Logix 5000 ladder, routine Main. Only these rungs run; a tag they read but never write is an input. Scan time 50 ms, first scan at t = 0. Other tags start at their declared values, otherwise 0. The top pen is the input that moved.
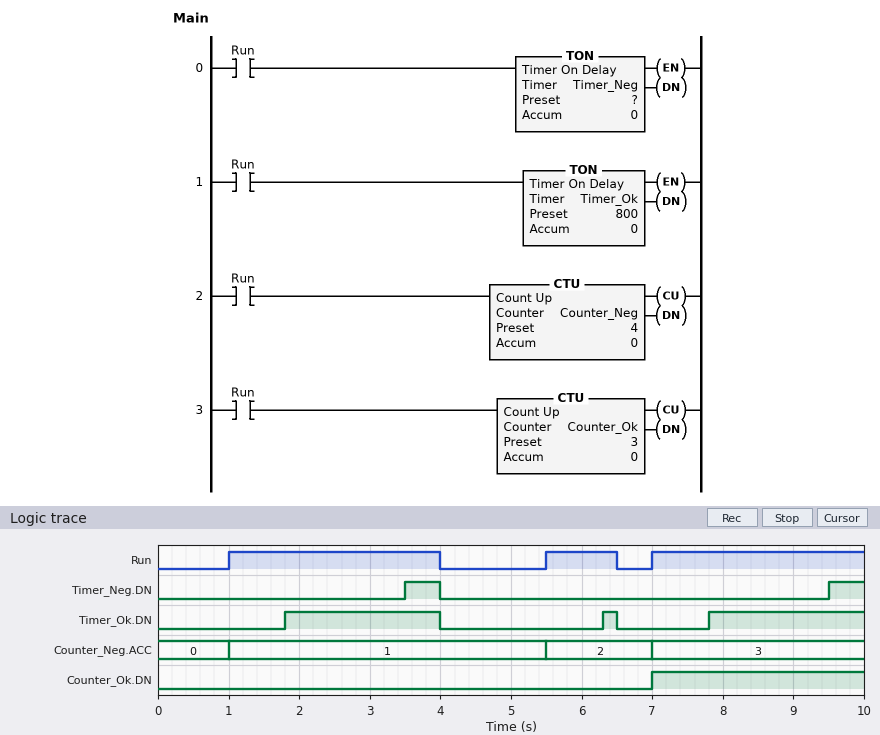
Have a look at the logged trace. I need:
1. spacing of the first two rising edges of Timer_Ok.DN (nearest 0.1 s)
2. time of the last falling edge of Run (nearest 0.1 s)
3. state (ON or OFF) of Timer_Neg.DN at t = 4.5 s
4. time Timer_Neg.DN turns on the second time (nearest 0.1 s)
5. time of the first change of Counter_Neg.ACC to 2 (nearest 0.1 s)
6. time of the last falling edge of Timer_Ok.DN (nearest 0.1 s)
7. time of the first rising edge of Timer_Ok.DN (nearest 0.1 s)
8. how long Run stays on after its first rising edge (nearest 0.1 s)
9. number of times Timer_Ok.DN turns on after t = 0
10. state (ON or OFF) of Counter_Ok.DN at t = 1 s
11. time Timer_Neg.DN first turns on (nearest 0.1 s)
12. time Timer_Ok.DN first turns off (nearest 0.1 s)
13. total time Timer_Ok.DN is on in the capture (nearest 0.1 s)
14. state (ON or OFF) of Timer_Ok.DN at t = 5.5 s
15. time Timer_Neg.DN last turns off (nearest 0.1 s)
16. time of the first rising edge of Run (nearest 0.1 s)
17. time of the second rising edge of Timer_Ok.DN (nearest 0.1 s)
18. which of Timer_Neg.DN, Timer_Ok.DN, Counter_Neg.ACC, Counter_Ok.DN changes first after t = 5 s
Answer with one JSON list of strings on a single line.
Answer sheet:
["4.5 s", "6.5 s", "OFF", "9.5 s", "5.5 s", "6.5 s", "1.8 s", "3.0 s", "3", "OFF", "3.5 s", "4.0 s", "4.6 s", "OFF", "4.0 s", "1.0 s", "6.3 s", "Counter_Neg.ACC"]
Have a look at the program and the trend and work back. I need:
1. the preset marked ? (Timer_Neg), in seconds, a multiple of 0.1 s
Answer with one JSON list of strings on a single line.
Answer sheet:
["2.5 s"]
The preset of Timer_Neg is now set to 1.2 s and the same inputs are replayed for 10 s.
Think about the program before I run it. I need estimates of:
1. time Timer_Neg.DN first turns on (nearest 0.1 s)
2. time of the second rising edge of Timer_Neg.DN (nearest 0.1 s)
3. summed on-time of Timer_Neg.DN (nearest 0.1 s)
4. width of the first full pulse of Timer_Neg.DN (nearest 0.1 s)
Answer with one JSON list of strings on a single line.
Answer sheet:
["2.2 s", "8.2 s", "3.6 s", "1.8 s"]
